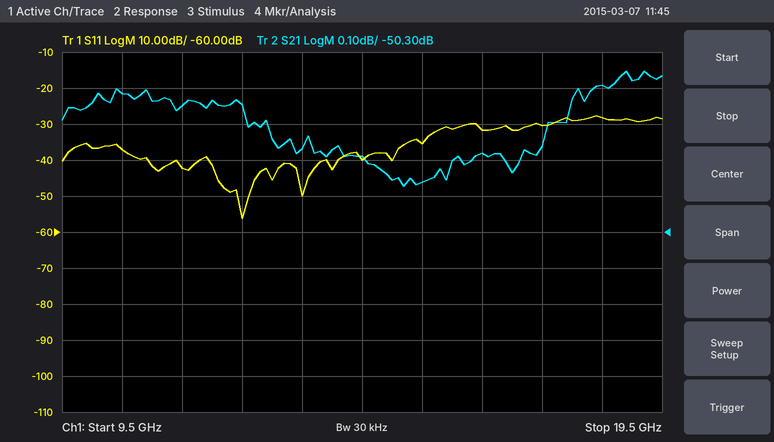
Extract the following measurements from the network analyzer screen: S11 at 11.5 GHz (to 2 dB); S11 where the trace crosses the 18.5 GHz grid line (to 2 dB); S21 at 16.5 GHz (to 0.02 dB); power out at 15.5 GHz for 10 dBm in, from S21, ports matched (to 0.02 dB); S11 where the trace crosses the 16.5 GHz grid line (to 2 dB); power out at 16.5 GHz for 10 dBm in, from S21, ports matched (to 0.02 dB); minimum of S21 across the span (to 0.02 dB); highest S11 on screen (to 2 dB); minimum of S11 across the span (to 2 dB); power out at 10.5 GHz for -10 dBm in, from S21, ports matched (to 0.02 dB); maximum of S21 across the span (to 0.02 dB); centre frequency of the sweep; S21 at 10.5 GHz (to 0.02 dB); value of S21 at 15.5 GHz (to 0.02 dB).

-42 dB
-28 dB
-50.08 dB
-40.16 dBm
-32 dB
-40.08 dBm
-50.18 dB
-28 dB
-56 dB
-59.92 dBm
-49.86 dB
14.5 GHz
-49.92 dB
-50.16 dB
